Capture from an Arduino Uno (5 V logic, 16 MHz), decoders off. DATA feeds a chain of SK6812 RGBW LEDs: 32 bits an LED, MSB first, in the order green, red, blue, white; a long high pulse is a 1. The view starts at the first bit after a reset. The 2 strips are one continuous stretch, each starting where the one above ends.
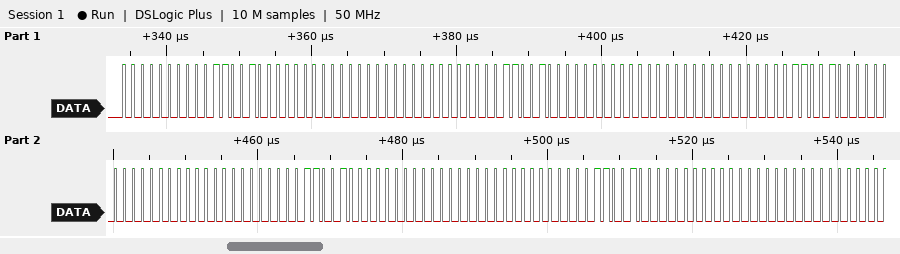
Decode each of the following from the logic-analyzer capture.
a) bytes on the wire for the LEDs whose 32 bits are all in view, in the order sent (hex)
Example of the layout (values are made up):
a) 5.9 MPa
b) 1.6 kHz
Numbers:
a) 00 32 00 00 00 32 00 00 00 32 00 00 00 32 00 00 00 32 00 00
